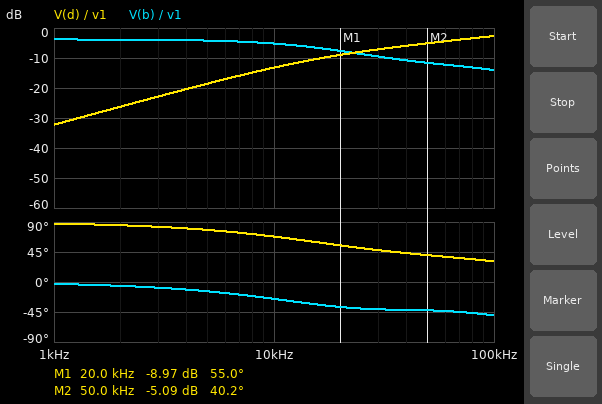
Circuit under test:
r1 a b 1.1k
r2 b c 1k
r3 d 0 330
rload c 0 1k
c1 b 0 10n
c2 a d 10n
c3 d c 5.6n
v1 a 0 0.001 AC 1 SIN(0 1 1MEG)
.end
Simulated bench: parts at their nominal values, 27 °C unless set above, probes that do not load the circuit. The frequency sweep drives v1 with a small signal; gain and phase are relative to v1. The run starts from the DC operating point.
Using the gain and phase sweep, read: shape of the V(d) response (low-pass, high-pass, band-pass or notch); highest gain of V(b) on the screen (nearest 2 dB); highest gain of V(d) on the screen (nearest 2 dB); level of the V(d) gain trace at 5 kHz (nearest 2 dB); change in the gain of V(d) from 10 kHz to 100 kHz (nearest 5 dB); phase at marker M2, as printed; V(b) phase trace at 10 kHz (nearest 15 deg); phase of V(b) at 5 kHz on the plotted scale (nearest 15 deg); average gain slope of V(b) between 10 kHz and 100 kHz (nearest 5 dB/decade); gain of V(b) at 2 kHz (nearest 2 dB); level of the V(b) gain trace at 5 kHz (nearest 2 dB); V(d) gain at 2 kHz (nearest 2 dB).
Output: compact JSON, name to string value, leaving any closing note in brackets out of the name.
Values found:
{"shape of the V(d) response": "high-pass", "highest gain of V(b) on the screen": "-4 dB", "highest gain of V(d) on the screen": "-2 dB", "level of the V(d) gain trace at 5 kHz": "-18 dB", "change in the gain of V(d) from 10 kHz to 100 kHz": "10 dB", "phase at marker M2, as printed": "40.2 deg", "V(b) phase trace at 10 kHz": "-30 deg", "phase of V(b) at 5 kHz on the plotted scale": "-15 deg", "average gain slope of V(b) between 10 kHz and 100 kHz": "-10 dB/decade", "gain of V(b) at 2 kHz": "-4 dB", "level of the V(b) gain trace at 5 kHz": "-4 dB", "V(d) gain at 2 kHz": "-26 dB"}
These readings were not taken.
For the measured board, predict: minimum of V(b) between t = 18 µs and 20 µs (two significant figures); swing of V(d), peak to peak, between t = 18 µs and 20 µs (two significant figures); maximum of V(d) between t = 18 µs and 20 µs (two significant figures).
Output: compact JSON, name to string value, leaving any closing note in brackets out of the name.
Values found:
{"minimum of V(b) between t = 18 µs and 20 µs": "-29 mV", "swing of V(d), peak to peak, between t = 18 µs and 20 µs": "2.0 V", "maximum of V(d) between t = 18 µs and 20 µs": "990 mV"}
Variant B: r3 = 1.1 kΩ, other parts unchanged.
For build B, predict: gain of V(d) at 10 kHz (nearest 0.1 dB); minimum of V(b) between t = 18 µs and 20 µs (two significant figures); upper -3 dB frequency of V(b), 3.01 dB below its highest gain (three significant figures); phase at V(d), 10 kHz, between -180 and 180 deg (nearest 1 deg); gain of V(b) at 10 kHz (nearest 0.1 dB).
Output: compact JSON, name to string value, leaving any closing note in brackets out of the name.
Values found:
{"gain of V(d) at 10 kHz": "-5.7 dB", "minimum of V(b) between t = 18 µs and 20 µs": "-29 mV", "upper -3 dB frequency of V(b), 3.01 dB below its highest gain": "18.8 kHz", "phase at V(d), 10 kHz, between -180 and 180 deg": "41 deg", "gain of V(b) at 10 kHz": "-5.3 dB"}
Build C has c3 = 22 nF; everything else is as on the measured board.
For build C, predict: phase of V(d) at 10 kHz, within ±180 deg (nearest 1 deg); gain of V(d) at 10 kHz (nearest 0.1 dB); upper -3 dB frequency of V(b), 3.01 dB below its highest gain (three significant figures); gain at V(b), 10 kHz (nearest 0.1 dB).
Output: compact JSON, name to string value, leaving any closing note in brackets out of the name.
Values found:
{"phase of V(d) at 10 kHz, within ±180 deg": "50 deg", "gain of V(d) at 10 kHz": "-13.8 dB", "upper -3 dB frequency of V(b), 3.01 dB below its highest gain": "13.9 kHz", "gain at V(b), 10 kHz": "-6.1 dB"}
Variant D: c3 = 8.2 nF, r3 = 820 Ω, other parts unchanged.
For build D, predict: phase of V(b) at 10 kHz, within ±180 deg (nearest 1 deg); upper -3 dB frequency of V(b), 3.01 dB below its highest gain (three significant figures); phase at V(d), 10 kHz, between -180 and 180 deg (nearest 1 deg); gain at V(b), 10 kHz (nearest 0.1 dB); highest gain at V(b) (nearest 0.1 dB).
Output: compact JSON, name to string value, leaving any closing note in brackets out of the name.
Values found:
{"phase of V(b) at 10 kHz, within ±180 deg": "-21 deg", "upper -3 dB frequency of V(b), 3.01 dB below its highest gain": "17.6 kHz", "phase at V(d), 10 kHz, between -180 and 180 deg": "44 deg", "gain at V(b), 10 kHz": "-5.5 dB", "highest gain at V(b)": "-3.8 dB"}
